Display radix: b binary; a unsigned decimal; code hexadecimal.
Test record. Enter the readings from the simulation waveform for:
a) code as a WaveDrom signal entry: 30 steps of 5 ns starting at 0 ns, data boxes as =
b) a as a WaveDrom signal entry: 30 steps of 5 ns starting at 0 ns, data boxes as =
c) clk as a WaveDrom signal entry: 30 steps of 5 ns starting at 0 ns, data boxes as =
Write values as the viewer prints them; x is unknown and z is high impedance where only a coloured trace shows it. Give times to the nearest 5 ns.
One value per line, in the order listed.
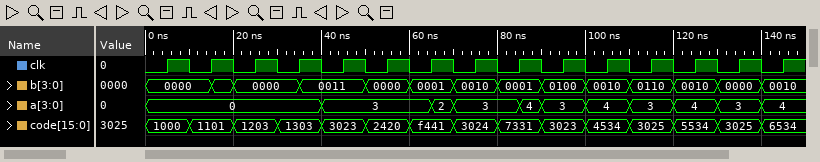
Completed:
{name: 'code', wave: '=.=.=.=.=.=.=.=.=.=.=.=.=.=.=.', data: '1000 1101 1203 1303 3023 2420 f441 3024 7331 3023 4534 3025 5534 3025 6534'}
{name: 'a', wave: '=.......=....==..==.=.=.=.=.=.', data: '0 3 2 3 4 3 4 3 4 3 4'}
{name: 'clk', wave: '010101010101010101010101010101'}
